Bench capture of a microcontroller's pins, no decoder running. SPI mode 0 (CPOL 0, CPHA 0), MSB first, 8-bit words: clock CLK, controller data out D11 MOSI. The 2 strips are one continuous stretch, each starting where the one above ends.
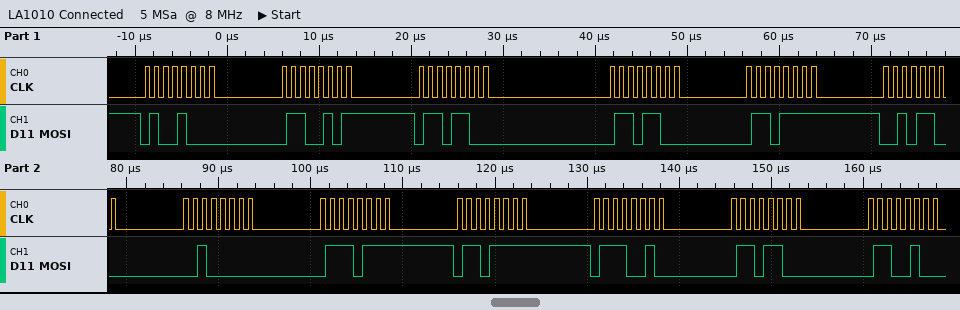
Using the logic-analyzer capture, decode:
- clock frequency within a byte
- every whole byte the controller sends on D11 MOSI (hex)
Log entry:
1 MHz
0x48 0x65 0x6C 0x6C 0x6F 0x2C 0x20 0x77 0x6F 0x72 0x6C 0x64
